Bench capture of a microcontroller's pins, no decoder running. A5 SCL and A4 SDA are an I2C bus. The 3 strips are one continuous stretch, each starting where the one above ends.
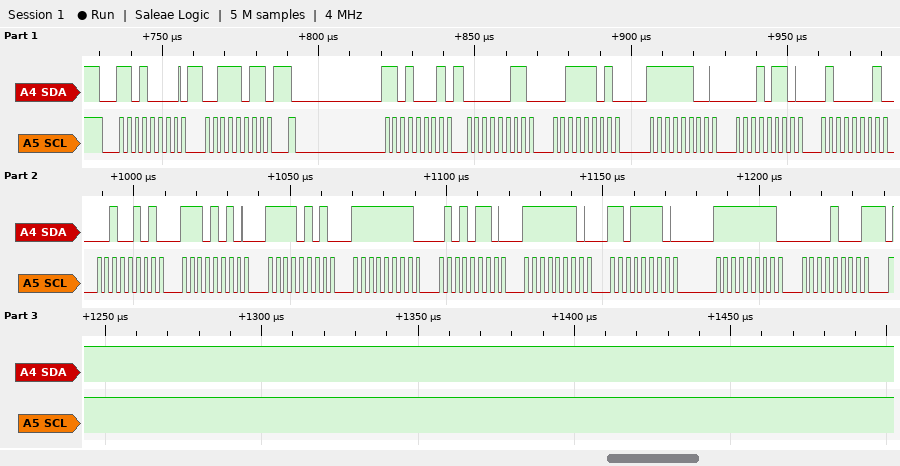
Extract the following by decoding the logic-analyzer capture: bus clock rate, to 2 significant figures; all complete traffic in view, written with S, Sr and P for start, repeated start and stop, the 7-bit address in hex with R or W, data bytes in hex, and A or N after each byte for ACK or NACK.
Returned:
400 kHz
S 68W A 3B A Sr 68R A 03 A 3D A FC A 16 A 41 A 25 A EA A F5 A FF A 56 A FE A DE A FF A 08 N P
